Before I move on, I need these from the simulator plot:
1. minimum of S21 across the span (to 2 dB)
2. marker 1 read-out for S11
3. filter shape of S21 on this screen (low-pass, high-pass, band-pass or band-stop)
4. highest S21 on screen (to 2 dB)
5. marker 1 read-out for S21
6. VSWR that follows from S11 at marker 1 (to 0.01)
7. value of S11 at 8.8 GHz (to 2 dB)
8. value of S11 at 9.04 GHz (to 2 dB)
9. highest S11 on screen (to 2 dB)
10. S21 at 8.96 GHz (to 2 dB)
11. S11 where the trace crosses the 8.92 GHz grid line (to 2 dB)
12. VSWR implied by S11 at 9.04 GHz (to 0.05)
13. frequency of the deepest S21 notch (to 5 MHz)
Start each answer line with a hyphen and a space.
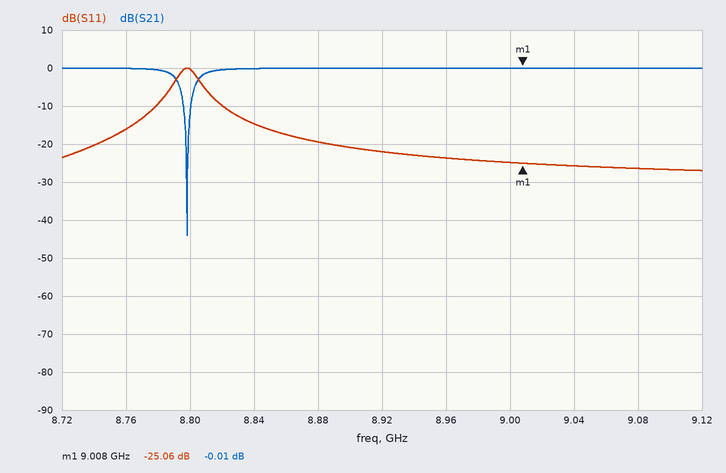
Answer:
- -44 dB
- -25.06 dB
- band-stop
- 0 dB
- -0.01 dB
- 1.12
- 0 dB
- -26 dB
- 0 dB
- 0 dB
- -22 dB
- 1.10
- 8.800 GHz
